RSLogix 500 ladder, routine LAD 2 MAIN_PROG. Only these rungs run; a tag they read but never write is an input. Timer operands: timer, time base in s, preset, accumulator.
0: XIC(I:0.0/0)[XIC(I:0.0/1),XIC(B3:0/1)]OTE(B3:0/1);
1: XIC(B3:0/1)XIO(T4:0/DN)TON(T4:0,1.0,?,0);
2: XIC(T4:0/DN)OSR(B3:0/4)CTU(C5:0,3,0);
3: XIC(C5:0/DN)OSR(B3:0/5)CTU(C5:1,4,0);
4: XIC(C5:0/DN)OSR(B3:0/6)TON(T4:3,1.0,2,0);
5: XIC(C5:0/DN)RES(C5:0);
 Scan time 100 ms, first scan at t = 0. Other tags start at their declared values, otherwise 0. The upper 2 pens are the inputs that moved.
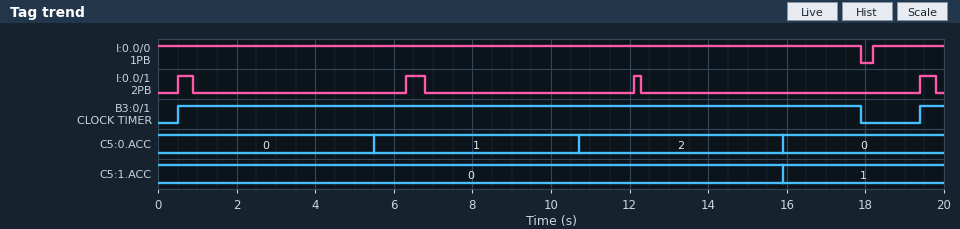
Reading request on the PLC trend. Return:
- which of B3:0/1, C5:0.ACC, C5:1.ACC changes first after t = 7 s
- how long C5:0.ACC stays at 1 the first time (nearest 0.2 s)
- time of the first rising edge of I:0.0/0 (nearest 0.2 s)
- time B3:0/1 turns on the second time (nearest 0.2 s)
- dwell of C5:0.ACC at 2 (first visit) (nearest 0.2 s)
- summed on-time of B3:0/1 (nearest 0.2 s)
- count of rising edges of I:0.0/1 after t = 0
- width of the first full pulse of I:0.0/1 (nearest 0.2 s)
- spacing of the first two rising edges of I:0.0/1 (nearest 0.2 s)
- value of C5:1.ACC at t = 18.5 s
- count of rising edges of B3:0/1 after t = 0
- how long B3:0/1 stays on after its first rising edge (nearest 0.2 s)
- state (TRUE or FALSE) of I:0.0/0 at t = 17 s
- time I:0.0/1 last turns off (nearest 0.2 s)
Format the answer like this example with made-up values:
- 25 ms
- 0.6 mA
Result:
- C5:0.ACC
- 5.2 s
- 18.2 s
- 19.4 s
- 5.2 s
- 18.0 s
- 4
- 0.4 s
- 5.8 s
- 1
- 2
- 17.4 s
- TRUE
- 19.8 s
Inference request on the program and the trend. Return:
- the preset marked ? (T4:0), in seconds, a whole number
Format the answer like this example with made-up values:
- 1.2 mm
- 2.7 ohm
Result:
- 5 s
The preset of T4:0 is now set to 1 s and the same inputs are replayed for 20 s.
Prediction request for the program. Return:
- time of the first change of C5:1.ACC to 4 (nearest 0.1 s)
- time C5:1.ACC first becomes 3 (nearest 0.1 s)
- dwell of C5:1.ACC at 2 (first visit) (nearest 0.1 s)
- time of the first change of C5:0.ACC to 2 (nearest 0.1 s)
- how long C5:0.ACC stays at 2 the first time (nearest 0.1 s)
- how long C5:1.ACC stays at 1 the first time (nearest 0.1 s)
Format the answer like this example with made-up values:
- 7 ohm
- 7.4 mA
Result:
- 14.7 s
- 11.1 s
- 3.6 s
- 2.7 s
- 1.2 s
- 3.6 s
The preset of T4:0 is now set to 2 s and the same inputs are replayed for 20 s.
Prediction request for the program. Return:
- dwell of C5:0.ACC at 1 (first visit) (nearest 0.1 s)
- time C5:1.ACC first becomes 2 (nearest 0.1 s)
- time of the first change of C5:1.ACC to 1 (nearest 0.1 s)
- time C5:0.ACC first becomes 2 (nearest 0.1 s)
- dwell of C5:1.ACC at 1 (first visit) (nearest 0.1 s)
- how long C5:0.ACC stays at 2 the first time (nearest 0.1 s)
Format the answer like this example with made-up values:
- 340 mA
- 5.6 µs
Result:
- 2.2 s
- 13.5 s
- 6.9 s
- 4.7 s
- 6.6 s
- 2.2 s
